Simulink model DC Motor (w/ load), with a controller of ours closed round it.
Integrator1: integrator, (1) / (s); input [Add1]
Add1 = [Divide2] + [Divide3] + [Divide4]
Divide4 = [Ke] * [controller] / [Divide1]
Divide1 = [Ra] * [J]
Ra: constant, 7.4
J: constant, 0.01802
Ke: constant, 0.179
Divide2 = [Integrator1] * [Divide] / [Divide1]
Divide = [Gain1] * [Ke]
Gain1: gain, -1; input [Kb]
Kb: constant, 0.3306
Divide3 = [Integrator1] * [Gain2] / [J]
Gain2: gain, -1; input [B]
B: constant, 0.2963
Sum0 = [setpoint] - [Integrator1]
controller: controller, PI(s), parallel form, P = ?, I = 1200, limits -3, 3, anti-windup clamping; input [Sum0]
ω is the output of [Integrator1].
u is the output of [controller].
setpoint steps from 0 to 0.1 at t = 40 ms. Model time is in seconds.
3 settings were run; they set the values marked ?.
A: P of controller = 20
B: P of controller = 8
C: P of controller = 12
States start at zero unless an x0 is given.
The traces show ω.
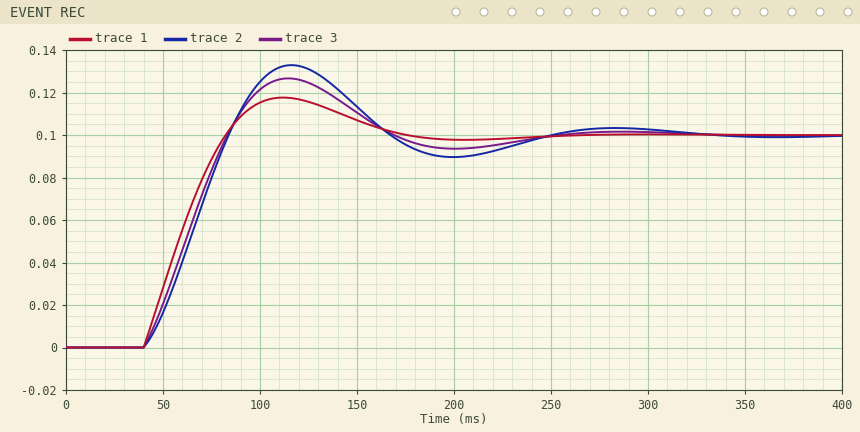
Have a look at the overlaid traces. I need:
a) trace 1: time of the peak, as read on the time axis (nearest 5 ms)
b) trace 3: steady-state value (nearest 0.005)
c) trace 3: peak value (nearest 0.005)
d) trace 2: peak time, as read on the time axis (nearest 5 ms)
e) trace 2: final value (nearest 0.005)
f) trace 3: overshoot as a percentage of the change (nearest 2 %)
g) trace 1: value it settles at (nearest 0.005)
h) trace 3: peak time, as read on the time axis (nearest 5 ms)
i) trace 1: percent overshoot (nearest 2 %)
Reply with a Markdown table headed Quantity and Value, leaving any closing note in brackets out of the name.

| Quantity | Value |
|---|---|
| trace 1: time of the peak, as read on the time axis | 110 ms |
| trace 3: steady-state value | 0.100 |
| trace 3: peak value | 0.125 |
| trace 2: peak time, as read on the time axis | 115 ms |
| trace 2: final value | 0.100 |
| trace 3: overshoot as a percentage of the change | 26 % |
| trace 1: value it settles at | 0.100 |
| trace 3: peak time, as read on the time axis | 115 ms |
| trace 1: percent overshoot | 18 % |
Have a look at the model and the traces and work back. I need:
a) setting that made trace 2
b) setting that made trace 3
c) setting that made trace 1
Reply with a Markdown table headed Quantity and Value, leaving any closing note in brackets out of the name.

| Quantity | Value |
|---|---|
| setting that made trace 2 | B |
| setting that made trace 3 | C |
| setting that made trace 1 | A |
